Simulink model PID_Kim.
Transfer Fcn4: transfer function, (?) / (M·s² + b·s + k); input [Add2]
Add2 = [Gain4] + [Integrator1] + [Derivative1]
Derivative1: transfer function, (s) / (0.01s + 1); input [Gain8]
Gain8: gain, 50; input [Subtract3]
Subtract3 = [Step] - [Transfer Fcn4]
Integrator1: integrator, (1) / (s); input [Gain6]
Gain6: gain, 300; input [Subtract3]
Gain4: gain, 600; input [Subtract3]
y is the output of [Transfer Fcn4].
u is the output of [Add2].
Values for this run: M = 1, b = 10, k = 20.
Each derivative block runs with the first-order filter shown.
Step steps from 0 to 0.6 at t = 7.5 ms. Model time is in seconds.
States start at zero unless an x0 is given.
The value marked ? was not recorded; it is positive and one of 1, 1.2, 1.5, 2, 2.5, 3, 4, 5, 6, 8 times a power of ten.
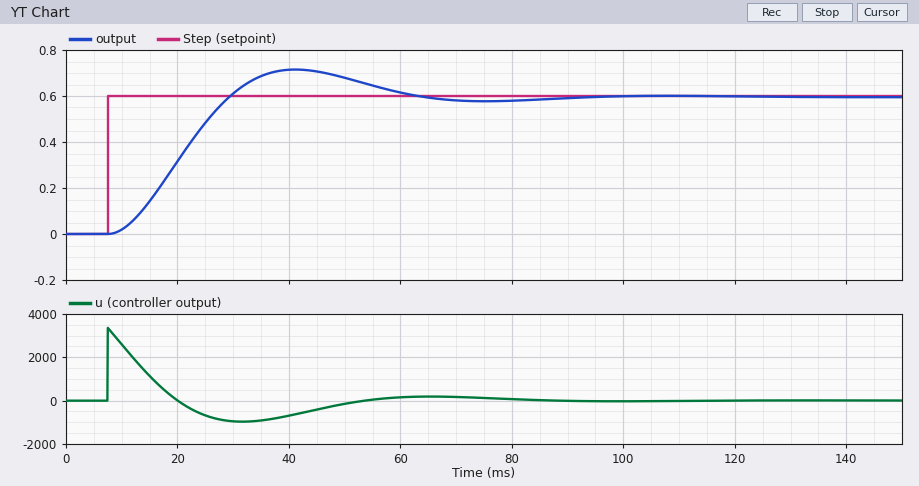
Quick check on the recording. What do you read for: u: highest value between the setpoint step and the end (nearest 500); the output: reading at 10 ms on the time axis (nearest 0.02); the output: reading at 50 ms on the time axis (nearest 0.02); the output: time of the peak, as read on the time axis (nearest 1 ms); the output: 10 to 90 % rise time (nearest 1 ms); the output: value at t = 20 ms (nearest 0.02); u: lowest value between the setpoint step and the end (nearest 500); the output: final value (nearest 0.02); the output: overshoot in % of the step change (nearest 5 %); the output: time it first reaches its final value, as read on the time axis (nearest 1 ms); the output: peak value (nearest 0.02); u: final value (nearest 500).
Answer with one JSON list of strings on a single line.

["3500", "0.02", "0.68", "41 ms", "15 ms", "0.32", "-1000", "0.60", "20 %", "29 ms", "0.72", "0"]
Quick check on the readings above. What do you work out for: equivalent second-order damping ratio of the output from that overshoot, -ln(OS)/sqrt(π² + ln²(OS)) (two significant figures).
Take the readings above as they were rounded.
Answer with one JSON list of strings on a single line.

["0.46"]
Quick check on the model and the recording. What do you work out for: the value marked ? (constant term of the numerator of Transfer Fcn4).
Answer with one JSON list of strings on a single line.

["2"]
